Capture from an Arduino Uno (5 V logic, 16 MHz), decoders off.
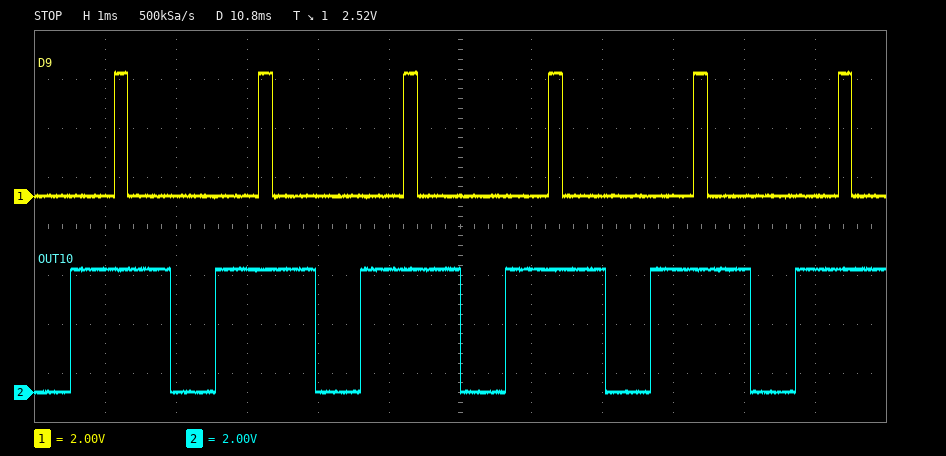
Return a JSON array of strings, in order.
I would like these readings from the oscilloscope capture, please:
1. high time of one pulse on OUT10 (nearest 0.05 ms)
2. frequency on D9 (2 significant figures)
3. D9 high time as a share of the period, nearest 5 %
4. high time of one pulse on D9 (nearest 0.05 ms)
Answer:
["1.40 ms", "490 Hz", "10 %", "0.20 ms"]
